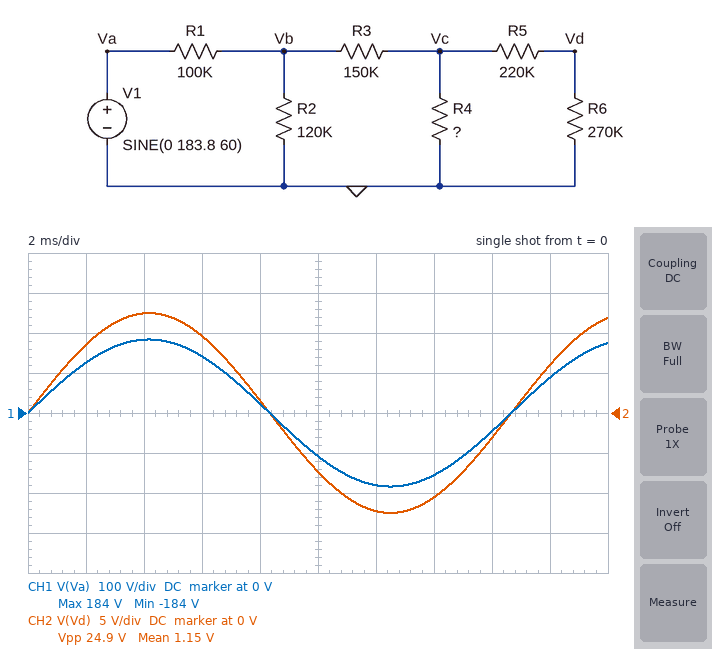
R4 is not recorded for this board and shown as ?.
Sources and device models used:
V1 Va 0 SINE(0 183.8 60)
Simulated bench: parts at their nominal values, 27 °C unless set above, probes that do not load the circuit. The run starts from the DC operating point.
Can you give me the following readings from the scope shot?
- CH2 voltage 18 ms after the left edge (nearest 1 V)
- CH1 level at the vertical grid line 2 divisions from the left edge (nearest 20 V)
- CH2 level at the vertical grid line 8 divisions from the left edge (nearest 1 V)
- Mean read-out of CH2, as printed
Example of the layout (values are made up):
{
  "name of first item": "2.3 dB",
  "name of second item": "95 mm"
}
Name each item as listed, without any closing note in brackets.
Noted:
{
  "CH2 voltage 18 ms after the left edge": "6 V",
  "CH1 level at the vertical grid line 2 divisions from the left edge": "180 V",
  "CH2 level at the vertical grid line 8 divisions from the left edge": "-3 V",
  "Mean read-out of CH2, as printed": "1.15 V"
}
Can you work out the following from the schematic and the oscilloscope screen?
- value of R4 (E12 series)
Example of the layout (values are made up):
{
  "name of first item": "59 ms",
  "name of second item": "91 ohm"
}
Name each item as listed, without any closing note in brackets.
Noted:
{
  "value of R4": "68 kΩ"
}
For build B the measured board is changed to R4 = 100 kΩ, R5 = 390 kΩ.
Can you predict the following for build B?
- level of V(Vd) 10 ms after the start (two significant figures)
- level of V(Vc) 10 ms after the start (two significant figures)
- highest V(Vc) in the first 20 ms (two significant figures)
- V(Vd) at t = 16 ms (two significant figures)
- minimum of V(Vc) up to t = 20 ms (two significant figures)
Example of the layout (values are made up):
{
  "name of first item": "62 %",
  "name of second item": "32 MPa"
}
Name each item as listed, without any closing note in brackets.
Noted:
{
  "level of V(Vd) 10 ms after the start": "-7.2 V",
  "level of V(Vc) 10 ms after the start": "-18 V",
  "highest V(Vc) in the first 20 ms": "30 V",
  "V(Vd) at t = 16 ms": "-3.0 V",
  "minimum of V(Vc) up to t = 20 ms": "-30 V"
}
